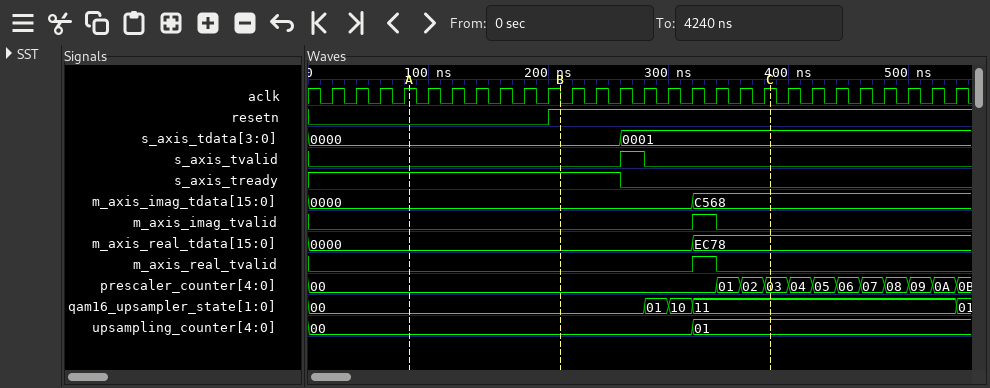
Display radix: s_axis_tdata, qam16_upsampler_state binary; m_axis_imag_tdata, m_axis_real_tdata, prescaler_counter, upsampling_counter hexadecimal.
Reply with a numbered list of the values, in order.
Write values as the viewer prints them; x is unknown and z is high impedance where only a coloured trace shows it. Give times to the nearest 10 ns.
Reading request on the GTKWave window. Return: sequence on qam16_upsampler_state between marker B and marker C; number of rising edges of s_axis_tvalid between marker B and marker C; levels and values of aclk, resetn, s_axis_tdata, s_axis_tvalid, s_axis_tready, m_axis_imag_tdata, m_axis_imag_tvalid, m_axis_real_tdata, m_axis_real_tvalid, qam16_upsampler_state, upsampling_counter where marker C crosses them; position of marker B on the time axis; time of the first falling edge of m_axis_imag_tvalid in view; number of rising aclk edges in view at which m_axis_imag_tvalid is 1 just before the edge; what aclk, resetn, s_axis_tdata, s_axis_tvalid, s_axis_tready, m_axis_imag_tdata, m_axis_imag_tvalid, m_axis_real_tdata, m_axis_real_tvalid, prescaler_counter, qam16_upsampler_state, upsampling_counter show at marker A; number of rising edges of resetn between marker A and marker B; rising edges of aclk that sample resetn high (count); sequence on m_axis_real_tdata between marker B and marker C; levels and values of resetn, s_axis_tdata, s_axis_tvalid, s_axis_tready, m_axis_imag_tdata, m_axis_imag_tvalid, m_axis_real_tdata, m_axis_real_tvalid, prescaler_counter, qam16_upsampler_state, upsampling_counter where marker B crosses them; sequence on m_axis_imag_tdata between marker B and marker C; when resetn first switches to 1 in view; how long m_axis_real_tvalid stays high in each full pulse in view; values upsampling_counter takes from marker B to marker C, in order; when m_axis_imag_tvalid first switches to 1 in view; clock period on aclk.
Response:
1. 00, 01, 10, 11
2. 1
3. aclk=1, resetn=1, s_axis_tdata=0001, s_axis_tvalid=0, s_axis_tready=0, m_axis_imag_tdata=C568, m_axis_imag_tvalid=0, m_axis_real_tdata=EC78, m_axis_real_tvalid=0, qam16_upsampler_state=11, upsampling_counter=01
4. 210 ns
5. 340 ns
6. 1
7. aclk=1, resetn=0, s_axis_tdata=0000, s_axis_tvalid=0, s_axis_tready=1, m_axis_imag_tdata=0000, m_axis_imag_tvalid=0, m_axis_real_tdata=0000, m_axis_real_tvalid=0, prescaler_counter=00, qam16_upsampler_state=00, upsampling_counter=00
8. 1
9. 17
10. 0000, EC78
11. resetn=1, s_axis_tdata=0000, s_axis_tvalid=0, s_axis_tready=1, m_axis_imag_tdata=0000, m_axis_imag_tvalid=0, m_axis_real_tdata=0000, m_axis_real_tvalid=0, prescaler_counter=00, qam16_upsampler_state=00, upsampling_counter=00
12. 0000, C568
13. 200 ns
14. 20 ns
15. 00, 01
16. 320 ns
17. 20 ns
